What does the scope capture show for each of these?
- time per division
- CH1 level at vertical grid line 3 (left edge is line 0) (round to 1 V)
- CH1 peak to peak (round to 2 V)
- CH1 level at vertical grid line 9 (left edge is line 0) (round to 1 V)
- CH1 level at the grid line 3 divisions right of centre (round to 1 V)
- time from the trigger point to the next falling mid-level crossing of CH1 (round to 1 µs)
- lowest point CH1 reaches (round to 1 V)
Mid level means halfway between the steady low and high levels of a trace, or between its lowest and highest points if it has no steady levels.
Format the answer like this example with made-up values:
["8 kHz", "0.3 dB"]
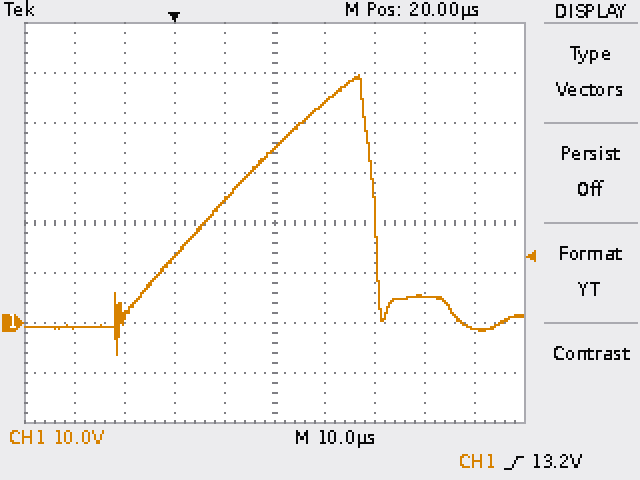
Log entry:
["10 µs", "13 V", "56 V", "-1 V", "5 V", "40 µs", "-6 V"]
